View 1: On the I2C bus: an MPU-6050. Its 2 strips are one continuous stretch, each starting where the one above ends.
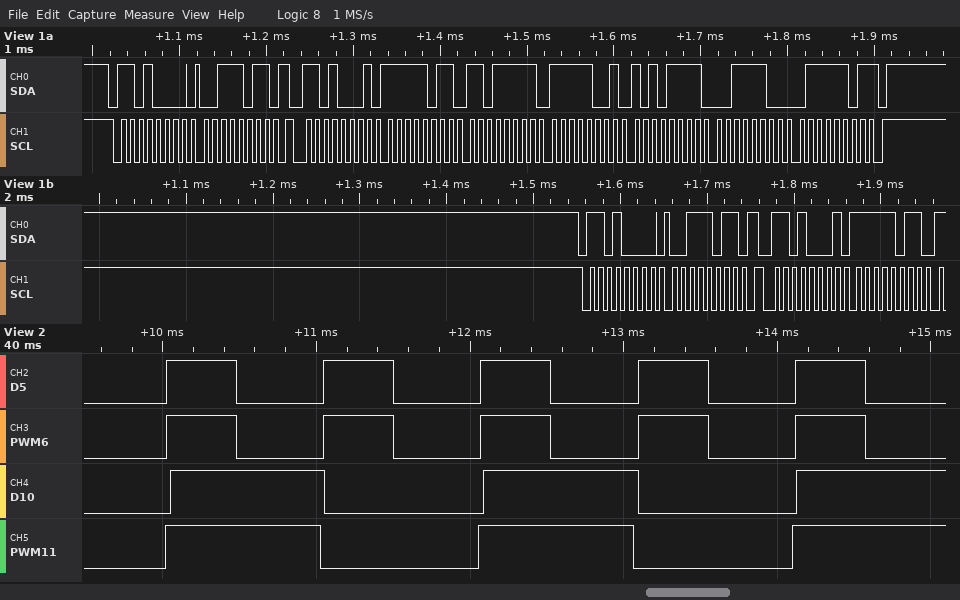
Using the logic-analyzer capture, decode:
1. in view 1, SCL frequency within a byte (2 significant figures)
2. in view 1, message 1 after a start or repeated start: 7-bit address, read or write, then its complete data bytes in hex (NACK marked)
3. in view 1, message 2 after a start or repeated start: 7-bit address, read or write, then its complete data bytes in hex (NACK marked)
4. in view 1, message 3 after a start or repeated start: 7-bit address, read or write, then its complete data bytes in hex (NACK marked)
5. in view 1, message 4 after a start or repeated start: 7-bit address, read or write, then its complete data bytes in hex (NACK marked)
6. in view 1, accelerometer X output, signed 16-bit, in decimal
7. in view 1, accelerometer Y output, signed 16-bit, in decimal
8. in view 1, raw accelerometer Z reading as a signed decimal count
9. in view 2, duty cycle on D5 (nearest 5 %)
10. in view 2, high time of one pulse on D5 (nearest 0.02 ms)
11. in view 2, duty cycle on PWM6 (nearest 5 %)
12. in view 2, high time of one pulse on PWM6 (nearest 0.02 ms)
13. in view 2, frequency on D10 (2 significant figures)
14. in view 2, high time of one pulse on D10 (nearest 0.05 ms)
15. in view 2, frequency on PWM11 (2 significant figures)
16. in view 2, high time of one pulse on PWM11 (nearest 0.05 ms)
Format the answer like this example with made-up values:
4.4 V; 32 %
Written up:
100 kHz; 0x68 write: 3B; 0x68 read: FB DF F9 AF 3C 7D NACK; 0x68 write: 3B; 0x68 read: FB; -1057; -1617; 15485; 45 %; 0.46 ms; 45 %; 0.46 ms; 490 Hz; 1.00 ms; 490 Hz; 1.00 ms
